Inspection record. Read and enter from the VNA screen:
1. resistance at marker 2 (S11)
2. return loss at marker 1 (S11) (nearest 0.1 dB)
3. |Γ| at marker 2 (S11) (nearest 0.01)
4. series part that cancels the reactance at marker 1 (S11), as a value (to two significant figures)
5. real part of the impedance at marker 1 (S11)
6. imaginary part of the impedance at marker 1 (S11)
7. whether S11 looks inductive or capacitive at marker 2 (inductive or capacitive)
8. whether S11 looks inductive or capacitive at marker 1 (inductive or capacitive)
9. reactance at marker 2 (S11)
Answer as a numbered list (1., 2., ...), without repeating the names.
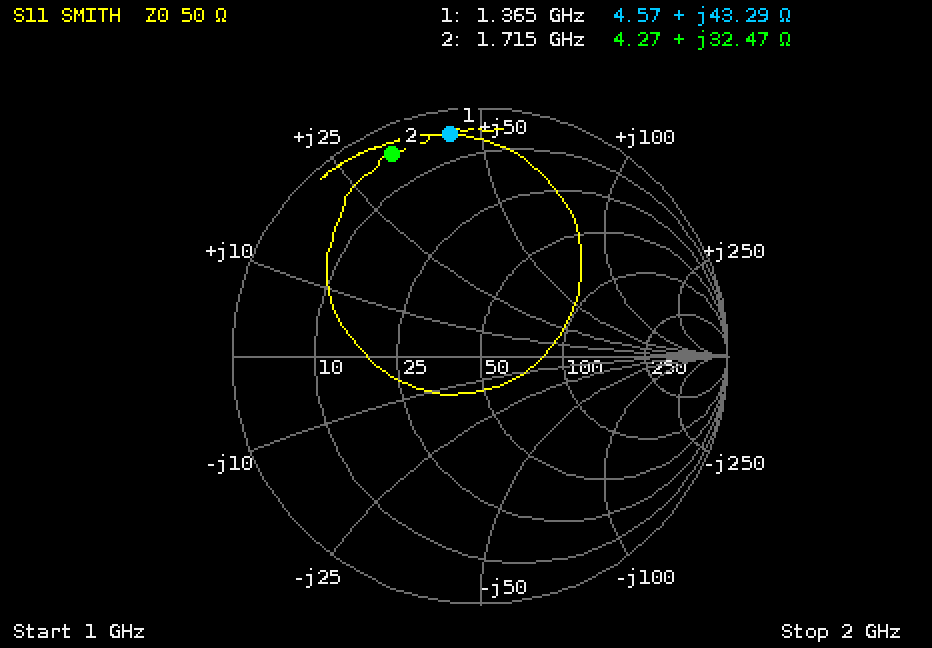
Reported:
1. 4.27 Ω
2. 0.9 dB
3. 0.89
4. 2.7 pF
5. 4.57 Ω
6. +43.29 Ω
7. inductive
8. inductive
9. +32.47 Ω
